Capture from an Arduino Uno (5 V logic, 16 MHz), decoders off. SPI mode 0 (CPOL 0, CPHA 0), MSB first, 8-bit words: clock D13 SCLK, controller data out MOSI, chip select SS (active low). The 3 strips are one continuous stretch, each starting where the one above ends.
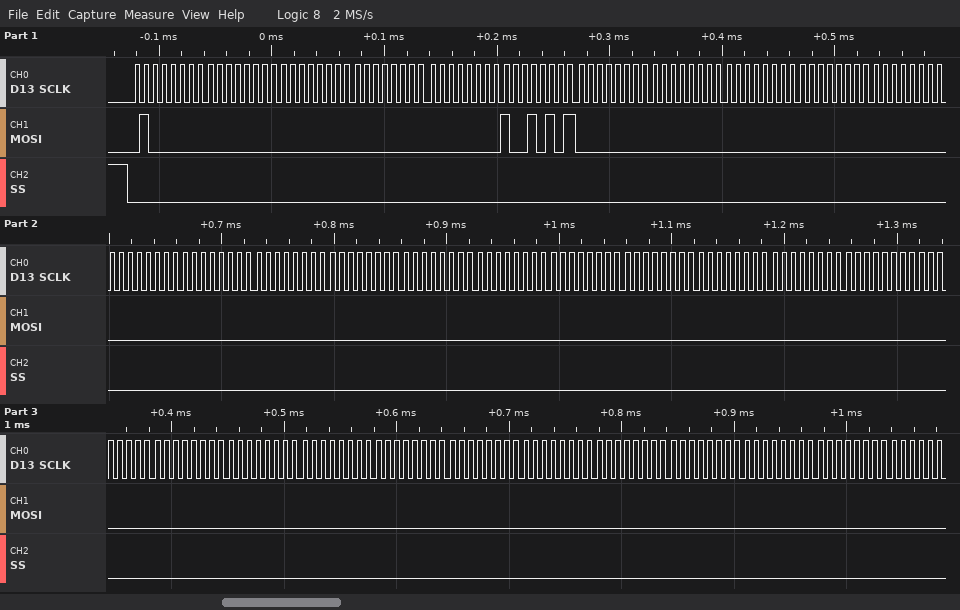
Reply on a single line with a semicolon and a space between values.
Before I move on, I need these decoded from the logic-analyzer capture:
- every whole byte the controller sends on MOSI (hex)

40 00 00 00 00 95 00 00 00 00 00 00 00 00 00 00 00 00 00 00 00 00 00 00 00 00 00 00 00 00 00 00 00
